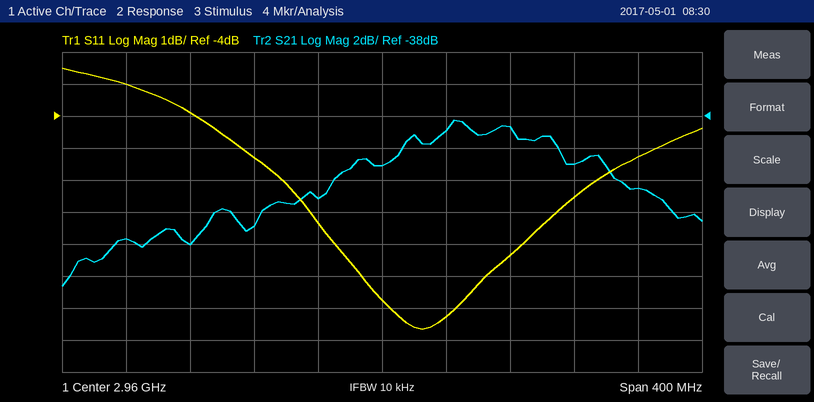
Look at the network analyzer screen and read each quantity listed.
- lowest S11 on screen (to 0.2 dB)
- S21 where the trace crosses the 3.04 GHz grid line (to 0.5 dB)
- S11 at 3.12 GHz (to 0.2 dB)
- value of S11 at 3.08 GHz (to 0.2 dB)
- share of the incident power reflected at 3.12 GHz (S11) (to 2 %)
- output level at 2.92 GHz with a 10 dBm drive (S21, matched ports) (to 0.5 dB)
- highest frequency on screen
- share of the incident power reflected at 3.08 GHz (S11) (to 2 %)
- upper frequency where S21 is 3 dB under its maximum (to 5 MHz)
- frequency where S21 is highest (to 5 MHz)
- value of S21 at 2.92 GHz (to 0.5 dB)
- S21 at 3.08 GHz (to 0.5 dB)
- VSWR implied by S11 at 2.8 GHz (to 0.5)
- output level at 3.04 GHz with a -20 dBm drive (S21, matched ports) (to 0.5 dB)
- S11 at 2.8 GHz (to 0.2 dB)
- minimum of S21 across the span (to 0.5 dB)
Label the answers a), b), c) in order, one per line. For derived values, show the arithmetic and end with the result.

a) -10.6 dB
b) -38.5 dB
c) -5.2 dB
d) -6.6 dB
e) 10^(-5.2/10) ≈ 30 %
f) 10 dBm + (-43.0 dB) = -33.0 dBm
g) 3.16 GHz
h) 10^(-6.6/10) ≈ 22 %
i) 3.100 GHz
j) 3.005 GHz
k) -43.0 dB
l) -41.0 dB
m) |Γ| = 10^(-3/20) = 0.7079; VSWR = (1 + 0.7079)/(1 − 0.7079) ≈ 5.85, so 6.0 to the nearest 0.5
n) -20 dBm + (-38.5 dB) = -58.5 dBm
o) -3.0 dB
p) -48.5 dB
